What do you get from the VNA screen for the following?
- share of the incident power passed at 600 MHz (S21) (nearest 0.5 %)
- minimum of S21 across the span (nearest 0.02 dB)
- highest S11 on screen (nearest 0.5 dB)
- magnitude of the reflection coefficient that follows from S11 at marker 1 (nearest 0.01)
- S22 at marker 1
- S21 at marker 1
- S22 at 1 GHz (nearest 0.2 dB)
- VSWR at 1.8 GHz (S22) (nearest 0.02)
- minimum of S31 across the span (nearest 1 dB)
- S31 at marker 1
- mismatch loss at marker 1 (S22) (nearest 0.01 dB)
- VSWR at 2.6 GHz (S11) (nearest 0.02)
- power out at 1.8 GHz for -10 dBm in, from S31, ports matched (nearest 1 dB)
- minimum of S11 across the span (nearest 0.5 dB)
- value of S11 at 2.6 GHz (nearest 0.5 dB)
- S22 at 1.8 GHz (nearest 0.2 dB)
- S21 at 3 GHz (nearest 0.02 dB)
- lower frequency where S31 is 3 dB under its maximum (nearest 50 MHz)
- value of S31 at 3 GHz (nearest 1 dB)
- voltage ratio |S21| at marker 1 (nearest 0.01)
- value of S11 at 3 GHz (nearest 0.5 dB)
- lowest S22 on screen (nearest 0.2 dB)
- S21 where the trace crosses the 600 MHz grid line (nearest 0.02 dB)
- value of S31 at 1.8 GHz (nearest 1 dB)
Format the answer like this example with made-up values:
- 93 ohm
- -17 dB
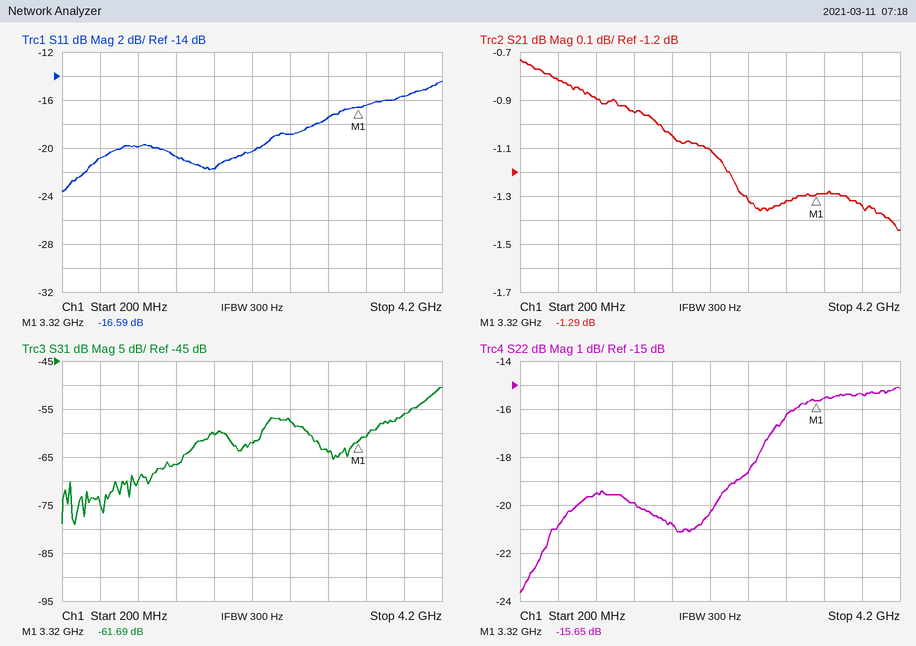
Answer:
- 83.0 %
- -1.44 dB
- -14.5 dB
- 0.15
- -15.65 dB
- -1.29 dB
- -19.6 dB
- 1.20
- -79 dB
- -61.69 dB
- 0.12 dB
- 1.26
- -70 dBm
- -23.5 dB
- -19.0 dB
- -20.8 dB
- -1.32 dB
- 4.00 GHz
- -64 dB
- 0.86
- -17.5 dB
- -23.6 dB
- -0.82 dB
- -60 dB
